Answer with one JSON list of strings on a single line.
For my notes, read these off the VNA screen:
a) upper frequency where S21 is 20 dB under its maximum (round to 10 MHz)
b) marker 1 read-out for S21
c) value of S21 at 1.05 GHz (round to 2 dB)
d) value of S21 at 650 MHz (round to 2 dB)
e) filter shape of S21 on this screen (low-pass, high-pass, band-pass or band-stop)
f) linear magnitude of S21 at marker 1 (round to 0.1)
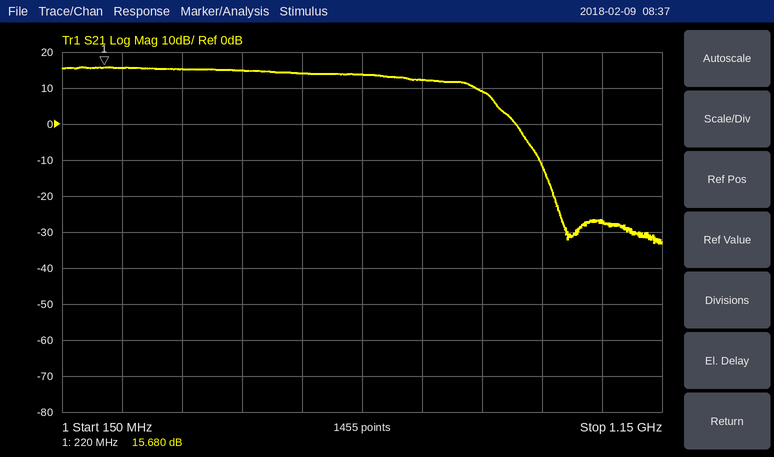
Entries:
["920 MHz", "15.680 dB", "-28 dB", "14 dB", "low-pass", "6.1"]
